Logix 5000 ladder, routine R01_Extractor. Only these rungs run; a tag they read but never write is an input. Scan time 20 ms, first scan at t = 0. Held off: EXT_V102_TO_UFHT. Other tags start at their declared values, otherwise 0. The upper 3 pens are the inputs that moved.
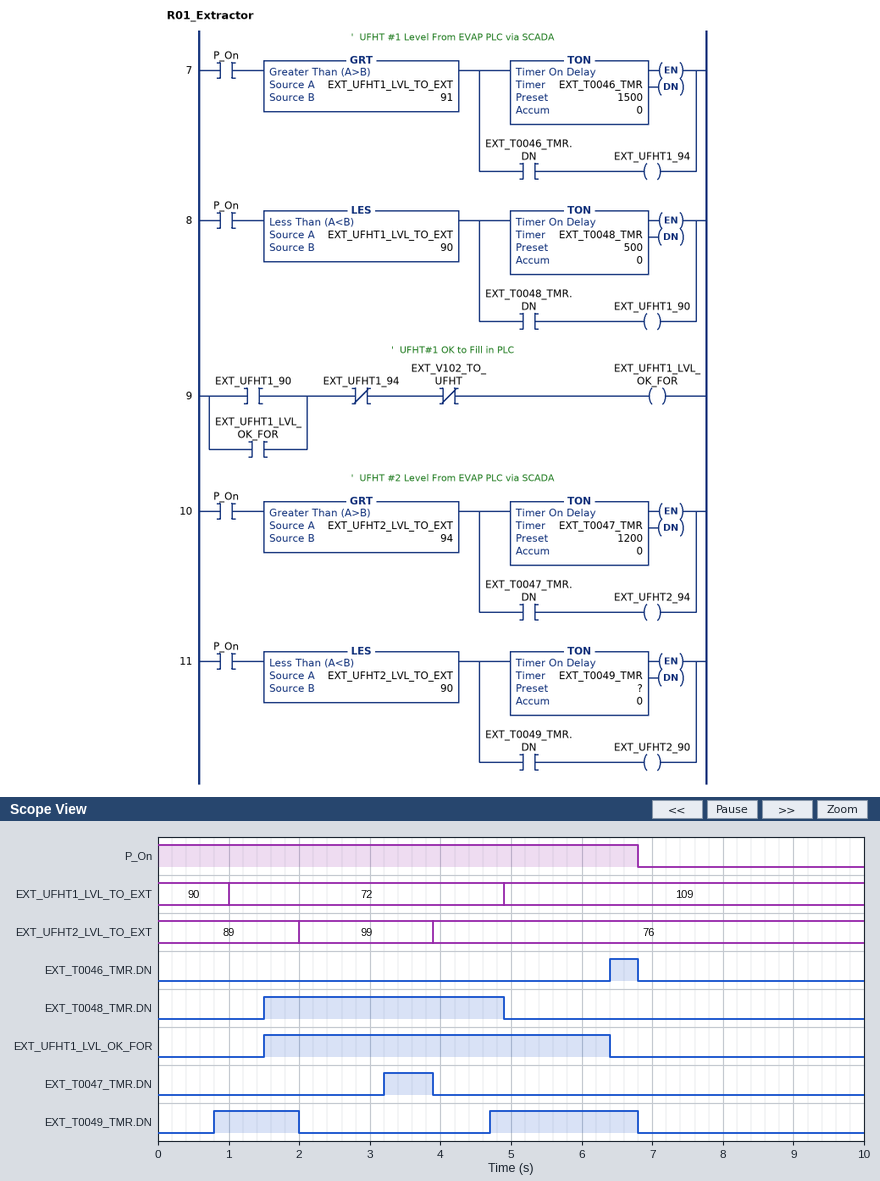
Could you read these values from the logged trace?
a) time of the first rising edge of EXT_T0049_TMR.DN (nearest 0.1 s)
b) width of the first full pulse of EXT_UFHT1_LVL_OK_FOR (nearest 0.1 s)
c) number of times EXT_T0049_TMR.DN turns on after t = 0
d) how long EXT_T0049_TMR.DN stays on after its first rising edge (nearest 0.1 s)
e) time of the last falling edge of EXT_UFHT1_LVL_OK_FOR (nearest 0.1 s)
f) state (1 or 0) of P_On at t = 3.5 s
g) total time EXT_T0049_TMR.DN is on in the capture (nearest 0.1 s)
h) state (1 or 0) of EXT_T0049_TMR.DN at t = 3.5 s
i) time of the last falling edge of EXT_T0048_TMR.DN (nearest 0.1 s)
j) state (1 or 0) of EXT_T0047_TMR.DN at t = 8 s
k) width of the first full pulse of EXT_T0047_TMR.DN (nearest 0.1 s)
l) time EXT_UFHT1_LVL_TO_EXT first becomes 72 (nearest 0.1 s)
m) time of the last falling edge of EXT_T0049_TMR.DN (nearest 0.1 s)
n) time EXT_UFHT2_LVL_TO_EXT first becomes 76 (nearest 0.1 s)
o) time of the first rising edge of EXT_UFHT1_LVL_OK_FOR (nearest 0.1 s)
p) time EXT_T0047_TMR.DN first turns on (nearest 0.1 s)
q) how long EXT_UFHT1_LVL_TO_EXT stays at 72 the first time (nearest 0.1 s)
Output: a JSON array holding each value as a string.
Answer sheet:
["0.8 s", "4.9 s", "2", "1.2 s", "6.4 s", "1", "3.3 s", "0", "4.9 s", "0", "0.7 s", "1.0 s", "6.8 s", "3.9 s", "1.5 s", "3.2 s", "3.9 s"]
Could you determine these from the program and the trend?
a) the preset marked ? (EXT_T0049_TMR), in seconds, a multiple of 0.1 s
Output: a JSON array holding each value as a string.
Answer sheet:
["0.8 s"]
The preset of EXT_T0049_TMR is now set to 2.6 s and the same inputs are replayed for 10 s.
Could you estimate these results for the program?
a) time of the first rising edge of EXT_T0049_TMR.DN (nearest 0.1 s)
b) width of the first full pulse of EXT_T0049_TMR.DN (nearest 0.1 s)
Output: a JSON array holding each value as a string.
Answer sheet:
["6.5 s", "0.3 s"]
